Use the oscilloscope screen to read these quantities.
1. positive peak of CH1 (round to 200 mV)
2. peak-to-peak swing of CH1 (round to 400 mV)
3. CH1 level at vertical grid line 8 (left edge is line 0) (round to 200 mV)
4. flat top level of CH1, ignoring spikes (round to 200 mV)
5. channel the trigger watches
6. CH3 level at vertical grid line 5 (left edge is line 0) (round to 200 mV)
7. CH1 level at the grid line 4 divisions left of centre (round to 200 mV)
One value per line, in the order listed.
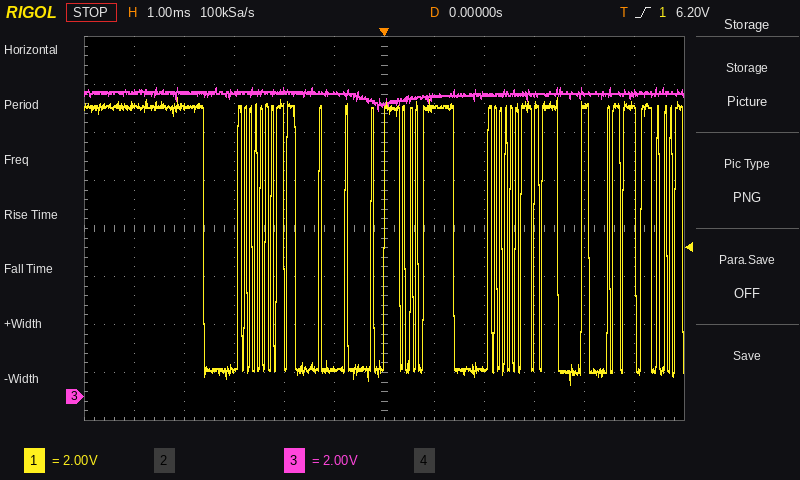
12.4 V
12.0 V
1.2 V
12.0 V
CH1
12.6 V
12.0 V
